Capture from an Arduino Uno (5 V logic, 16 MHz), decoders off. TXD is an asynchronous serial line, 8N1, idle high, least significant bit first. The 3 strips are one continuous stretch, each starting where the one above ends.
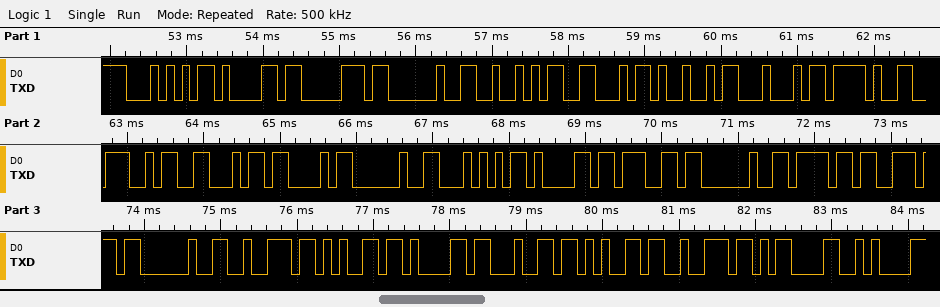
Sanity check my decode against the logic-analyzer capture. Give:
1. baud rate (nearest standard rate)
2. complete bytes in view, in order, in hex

9600 baud
54 61 70 20 52 46 49 44 2F 4E 46 43 20 54 61 67 20 6F 6E 20 72 65 61 64 65 72 0D 0A
